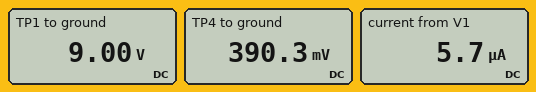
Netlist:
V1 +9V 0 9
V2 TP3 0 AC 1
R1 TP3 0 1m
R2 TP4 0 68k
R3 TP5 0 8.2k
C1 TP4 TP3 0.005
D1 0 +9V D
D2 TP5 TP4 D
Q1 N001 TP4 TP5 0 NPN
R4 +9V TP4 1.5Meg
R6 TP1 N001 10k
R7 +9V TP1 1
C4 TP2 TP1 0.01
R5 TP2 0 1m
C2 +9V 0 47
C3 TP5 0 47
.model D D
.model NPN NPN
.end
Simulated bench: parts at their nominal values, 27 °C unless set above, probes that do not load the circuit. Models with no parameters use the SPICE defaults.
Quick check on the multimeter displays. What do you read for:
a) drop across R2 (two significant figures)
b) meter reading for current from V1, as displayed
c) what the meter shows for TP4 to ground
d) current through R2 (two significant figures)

390 mV
5.7 µA
390.3 mV
5.7 µA
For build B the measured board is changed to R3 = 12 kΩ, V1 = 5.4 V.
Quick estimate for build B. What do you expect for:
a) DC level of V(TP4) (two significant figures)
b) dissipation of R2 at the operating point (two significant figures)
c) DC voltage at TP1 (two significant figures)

230 mV
810 nW
5.4 V
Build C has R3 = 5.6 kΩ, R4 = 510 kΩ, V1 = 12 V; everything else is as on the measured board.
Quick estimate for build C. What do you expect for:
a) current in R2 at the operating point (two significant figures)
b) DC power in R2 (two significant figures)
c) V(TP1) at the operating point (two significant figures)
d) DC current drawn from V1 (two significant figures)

20 µA
27 µW
12 V
130 µA
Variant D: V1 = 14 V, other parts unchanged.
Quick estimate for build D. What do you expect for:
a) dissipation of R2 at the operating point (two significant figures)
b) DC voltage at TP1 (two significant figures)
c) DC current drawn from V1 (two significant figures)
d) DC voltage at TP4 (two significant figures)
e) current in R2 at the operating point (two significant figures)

5.4 µW
14 V
10 µA
610 mV
8.9 µA
